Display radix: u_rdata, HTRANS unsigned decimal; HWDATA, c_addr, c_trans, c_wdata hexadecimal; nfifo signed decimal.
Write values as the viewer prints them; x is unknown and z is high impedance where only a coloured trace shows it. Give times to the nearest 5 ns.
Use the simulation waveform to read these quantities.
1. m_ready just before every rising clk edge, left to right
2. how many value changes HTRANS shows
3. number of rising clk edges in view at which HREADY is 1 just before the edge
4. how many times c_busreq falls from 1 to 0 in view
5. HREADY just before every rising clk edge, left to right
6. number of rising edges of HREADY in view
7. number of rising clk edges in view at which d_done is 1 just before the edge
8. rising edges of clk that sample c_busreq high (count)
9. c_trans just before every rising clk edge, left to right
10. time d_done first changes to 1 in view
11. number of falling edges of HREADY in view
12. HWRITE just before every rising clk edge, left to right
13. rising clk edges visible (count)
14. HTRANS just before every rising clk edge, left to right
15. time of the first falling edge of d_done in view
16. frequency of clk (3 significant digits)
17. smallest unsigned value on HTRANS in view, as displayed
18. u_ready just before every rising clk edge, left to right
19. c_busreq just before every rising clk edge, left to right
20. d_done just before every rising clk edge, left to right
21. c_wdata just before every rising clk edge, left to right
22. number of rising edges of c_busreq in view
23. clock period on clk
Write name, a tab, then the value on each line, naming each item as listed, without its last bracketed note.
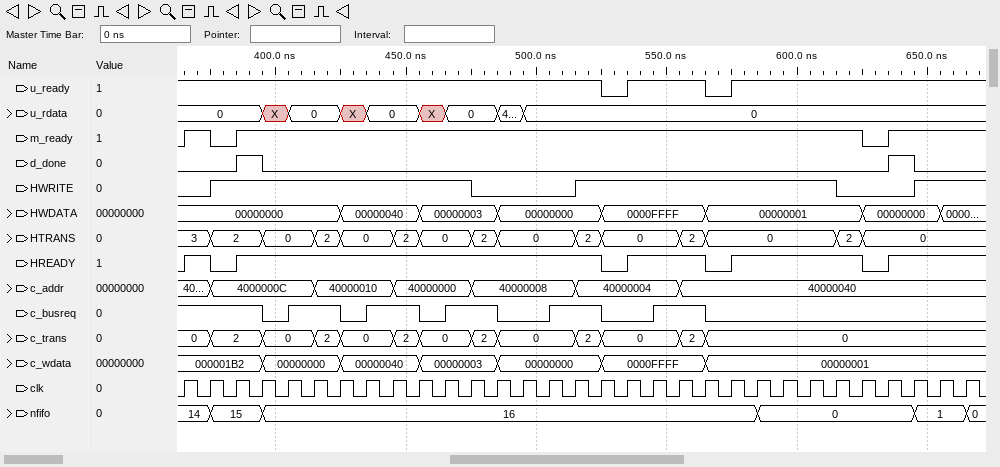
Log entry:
m_ready just before every rising clk edge, left to right	0 1 0 1 1 1 1 1 1 1 1 1 1 1 1 1 1 1 1 1 1 1 1 1 1 1 1 0 1 1 1
how many value changes HTRANS shows	14
number of rising clk edges in view at which HREADY is 1 just before the edge	26
how many times c_busreq falls from 1 to 0 in view	6
HREADY just before every rising clk edge, left to right	0 1 0 1 1 1 1 1 1 1 1 1 1 1 1 1 1 0 1 1 1 0 1 1 1 1 1 0 1 1 1
number of rising edges of HREADY in view	5
number of rising clk edges in view at which d_done is 1 just before the edge	2
rising edges of clk that sample c_busreq high	14
c_trans just before every rising clk edge, left to right	0, 0, 2, 2, 0, 0, 2, 0, 0, 2, 0, 0, 2, 0, 0, 0, 2, 0, 0, 0, 2, 0, 0, 0, 0, 0, 0, 0, 0, 0, 0
time d_done first changes to 1 in view	385 ns
number of falling edges of HREADY in view	4
HWRITE just before every rising clk edge, left to right	0 0 1 1 1 1 1 1 1 1 1 1 0 0 0 0 1 1 1 1 1 1 1 1 1 1 0 0 0 1 1
rising clk edges visible	31
HTRANS just before every rising clk edge, left to right	3, 3, 2, 2, 0, 0, 2, 0, 0, 2, 0, 0, 2, 0, 0, 0, 2, 0, 0, 0, 2, 0, 0, 0, 0, 0, 2, 0, 0, 0, 0
time of the first falling edge of d_done in view	395 ns
frequency of clk	100 MHz
smallest unsigned value on HTRANS in view, as displayed	0
u_ready just before every rising clk edge, left to right	1 1 1 1 1 1 1 1 1 1 1 1 1 1 1 1 1 0 1 1 1 0 1 1 1 1 1 1 1 1 1
c_busreq just before every rising clk edge, left to right	1 1 1 1 0 1 1 0 1 1 0 1 1 0 0 1 1 0 0 1 1 0 0 0 0 0 0 0 0 0 0
d_done just before every rising clk edge, left to right	0 0 0 1 0 0 0 0 0 0 0 0 0 0 0 0 0 0 0 0 0 0 0 0 0 0 0 0 1 0 0
c_wdata just before every rising clk edge, left to right	000001B2, 000001B2, 000001B2, 000001B2, 00000000, 00000000, 00000000, 00000040, 00000040, 00000040, 00000003, 00000003, 00000003, 00000000, 00000000, 00000000, 00000000, 0000FFFF, 0000FFFF, 0000FFFF, 0000FFFF, 00000001, 00000001, 00000001, 00000001, 00000001, 00000001, 00000001, 00000001, 00000001, 00000001
number of rising edges of c_busreq in view	5
clock period on clk	10 ns
